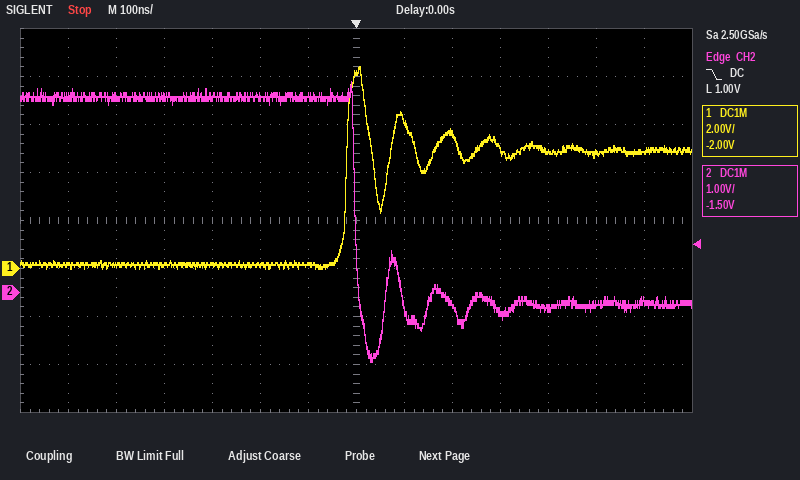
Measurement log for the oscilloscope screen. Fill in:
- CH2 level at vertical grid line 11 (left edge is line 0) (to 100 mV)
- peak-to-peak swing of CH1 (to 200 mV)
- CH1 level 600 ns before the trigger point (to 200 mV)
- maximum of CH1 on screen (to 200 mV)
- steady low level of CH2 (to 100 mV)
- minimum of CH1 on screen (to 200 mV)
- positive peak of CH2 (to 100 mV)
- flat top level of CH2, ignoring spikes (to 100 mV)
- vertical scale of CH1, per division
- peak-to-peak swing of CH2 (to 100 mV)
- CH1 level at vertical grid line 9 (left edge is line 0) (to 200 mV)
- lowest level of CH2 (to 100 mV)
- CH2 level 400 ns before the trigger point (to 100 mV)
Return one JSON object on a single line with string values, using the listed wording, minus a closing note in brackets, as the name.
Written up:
{"CH2 level at vertical grid line 11 (left edge is line 0)": "-300 mV", "peak-to-peak swing of CH1": "8.4 V", "CH1 level 600 ns before the trigger point": "200 mV", "maximum of CH1 on screen": "8.4 V", "steady low level of CH2": "-200 mV", "minimum of CH1 on screen": "0.0 V", "positive peak of CH2": "4.4 V", "flat top level of CH2, ignoring spikes": "4.1 V", "vertical scale of CH1, per division": "2 V", "peak-to-peak swing of CH2": "5.8 V", "CH1 level at vertical grid line 9 (left edge is line 0)": "5.6 V", "lowest level of CH2": "-1.4 V", "CH2 level 400 ns before the trigger point": "4.1 V"}
